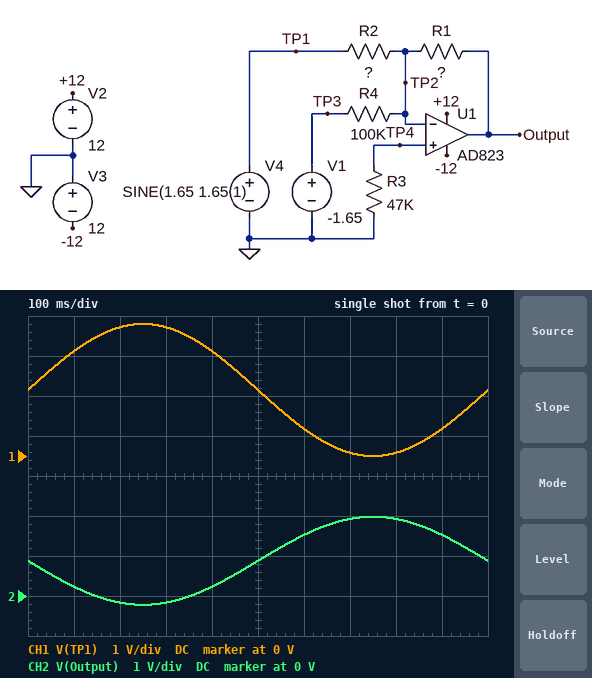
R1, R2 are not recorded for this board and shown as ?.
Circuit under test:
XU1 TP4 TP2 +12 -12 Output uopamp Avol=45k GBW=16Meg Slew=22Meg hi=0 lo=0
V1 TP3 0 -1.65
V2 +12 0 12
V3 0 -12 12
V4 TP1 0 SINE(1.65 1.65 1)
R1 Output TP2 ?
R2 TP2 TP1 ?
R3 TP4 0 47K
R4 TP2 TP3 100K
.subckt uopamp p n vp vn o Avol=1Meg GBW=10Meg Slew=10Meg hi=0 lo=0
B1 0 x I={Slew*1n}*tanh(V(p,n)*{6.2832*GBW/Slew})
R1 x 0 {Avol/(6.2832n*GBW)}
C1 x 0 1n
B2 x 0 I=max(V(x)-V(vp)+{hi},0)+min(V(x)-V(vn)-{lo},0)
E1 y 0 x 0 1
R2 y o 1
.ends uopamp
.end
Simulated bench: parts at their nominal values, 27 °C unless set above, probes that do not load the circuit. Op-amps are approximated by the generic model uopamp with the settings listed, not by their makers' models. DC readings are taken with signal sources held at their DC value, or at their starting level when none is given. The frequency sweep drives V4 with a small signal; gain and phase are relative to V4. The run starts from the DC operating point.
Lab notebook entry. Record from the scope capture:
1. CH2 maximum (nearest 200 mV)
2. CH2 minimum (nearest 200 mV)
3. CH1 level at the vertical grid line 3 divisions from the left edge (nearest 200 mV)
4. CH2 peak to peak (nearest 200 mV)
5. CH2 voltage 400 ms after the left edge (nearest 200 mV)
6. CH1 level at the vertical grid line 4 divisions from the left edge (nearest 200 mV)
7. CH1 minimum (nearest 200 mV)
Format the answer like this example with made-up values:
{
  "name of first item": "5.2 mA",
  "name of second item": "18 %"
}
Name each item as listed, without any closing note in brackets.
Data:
{
  "CH2 maximum": "2.0 V",
  "CH2 minimum": "-200 mV",
  "CH1 level at the vertical grid line 3 divisions from the left edge": "3.2 V",
  "CH2 peak to peak": "2.2 V",
  "CH2 voltage 400 ms after the left edge": "200 mV",
  "CH1 level at the vertical grid line 4 divisions from the left edge": "2.6 V",
  "CH1 minimum": "0 V"
}
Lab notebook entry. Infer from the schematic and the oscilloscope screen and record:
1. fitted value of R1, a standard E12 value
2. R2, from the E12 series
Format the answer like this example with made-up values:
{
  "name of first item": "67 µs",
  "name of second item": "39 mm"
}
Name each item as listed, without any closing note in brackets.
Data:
{
  "fitted value of R1, a standard E12 value": "120 kΩ",
  "R2, from the E12 series": "180 kΩ"
}
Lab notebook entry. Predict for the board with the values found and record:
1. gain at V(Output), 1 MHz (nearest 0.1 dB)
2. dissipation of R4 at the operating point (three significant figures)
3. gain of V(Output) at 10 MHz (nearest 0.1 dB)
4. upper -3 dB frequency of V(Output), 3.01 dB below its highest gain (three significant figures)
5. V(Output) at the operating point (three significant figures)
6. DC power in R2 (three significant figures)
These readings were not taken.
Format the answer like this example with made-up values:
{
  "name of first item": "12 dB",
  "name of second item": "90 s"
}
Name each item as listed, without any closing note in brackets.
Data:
{
  "gain at V(Output), 1 MHz": "-3.7 dB",
  "dissipation of R4 at the operating point": "27.2 µW",
  "gain of V(Output) at 10 MHz": "-9.8 dB",
  "upper -3 dB frequency of V(Output), 3.01 dB below its highest gain": "5.58 MHz",
  "V(Output) at the operating point": "880 mV",
  "DC power in R2": "15.1 µW"
}
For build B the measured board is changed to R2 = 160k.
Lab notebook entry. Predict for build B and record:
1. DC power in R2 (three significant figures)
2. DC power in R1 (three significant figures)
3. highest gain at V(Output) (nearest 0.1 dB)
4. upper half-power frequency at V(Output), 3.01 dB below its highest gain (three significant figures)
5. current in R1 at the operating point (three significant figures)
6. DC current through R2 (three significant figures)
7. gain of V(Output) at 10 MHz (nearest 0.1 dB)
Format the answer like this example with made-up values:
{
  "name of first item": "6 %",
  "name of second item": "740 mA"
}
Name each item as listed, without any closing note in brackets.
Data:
{
  "DC power in R2": "17.0 µW",
  "DC power in R1": "4.59 µW",
  "highest gain at V(Output)": "-2.5 dB",
  "upper half-power frequency at V(Output), 3.01 dB below its highest gain": "5.42 MHz",
  "current in R1 at the operating point": "6.19 µA",
  "DC current through R2": "10.3 µA",
  "gain of V(Output) at 10 MHz": "-8.9 dB"
}
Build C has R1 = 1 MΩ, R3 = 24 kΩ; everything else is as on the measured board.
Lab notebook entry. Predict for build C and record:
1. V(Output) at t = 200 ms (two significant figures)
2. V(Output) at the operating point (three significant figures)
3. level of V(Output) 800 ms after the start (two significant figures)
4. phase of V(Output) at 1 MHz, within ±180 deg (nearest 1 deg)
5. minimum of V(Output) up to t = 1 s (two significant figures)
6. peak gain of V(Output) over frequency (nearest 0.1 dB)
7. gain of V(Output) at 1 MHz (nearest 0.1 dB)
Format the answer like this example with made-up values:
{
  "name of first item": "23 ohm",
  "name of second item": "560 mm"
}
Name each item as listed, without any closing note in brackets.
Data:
{
  "V(Output) at t = 200 ms": "-1.4 V",
  "V(Output) at the operating point": "7.33 V",
  "level of V(Output) 800 ms after the start": "12 V",
  "phase of V(Output) at 1 MHz, within ±180 deg": "134 deg",
  "minimum of V(Output) up to t = 1 s": "-1.8 V",
  "peak gain of V(Output) over frequency": "14.9 dB",
  "gain of V(Output) at 1 MHz": "11.7 dB"
}
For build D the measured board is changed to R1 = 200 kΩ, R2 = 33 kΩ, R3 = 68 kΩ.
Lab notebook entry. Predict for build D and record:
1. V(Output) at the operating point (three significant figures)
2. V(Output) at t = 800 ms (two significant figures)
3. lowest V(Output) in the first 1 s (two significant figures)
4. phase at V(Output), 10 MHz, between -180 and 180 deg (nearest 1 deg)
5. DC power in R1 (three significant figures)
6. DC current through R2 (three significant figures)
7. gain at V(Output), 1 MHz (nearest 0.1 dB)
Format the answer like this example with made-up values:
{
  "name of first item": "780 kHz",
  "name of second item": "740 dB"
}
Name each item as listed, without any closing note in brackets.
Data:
{
  "V(Output) at the operating point": "-6.70 V",
  "V(Output) at t = 800 ms": "2.8 V",
  "lowest V(Output) in the first 1 s": "-12 V",
  "phase at V(Output), 10 MHz, between -180 and 180 deg": "100 deg",
  "DC power in R1": "224 µW",
  "DC current through R2": "50.0 µA",
  "gain at V(Output), 1 MHz": "14.4 dB"
}
